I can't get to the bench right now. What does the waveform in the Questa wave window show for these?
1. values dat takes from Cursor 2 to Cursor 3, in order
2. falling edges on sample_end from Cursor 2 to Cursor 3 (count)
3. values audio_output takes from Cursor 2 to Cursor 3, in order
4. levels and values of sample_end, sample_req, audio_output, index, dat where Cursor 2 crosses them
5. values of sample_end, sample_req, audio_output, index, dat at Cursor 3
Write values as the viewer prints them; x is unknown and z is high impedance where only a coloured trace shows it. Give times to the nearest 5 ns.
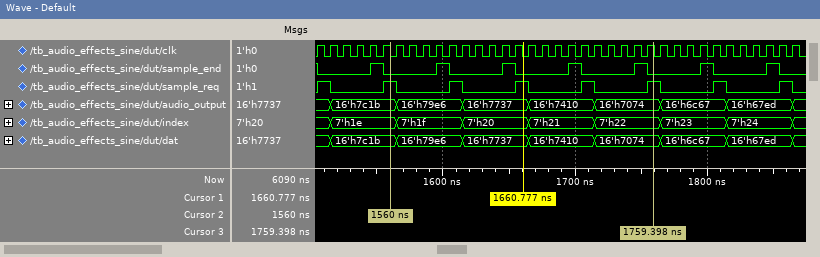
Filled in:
16'h7c1b, 16'h79e6, 16'h7737, 16'h7410, 16'h7074
4
16'h7c1b, 16'h79e6, 16'h7737, 16'h7410, 16'h7074
sample_end=0, sample_req=1, audio_output=16'h7c1b, index=7'h1e, dat=16'h7c1b
sample_end=0, sample_req=1, audio_output=16'h7074, index=7'h22, dat=16'h7074
